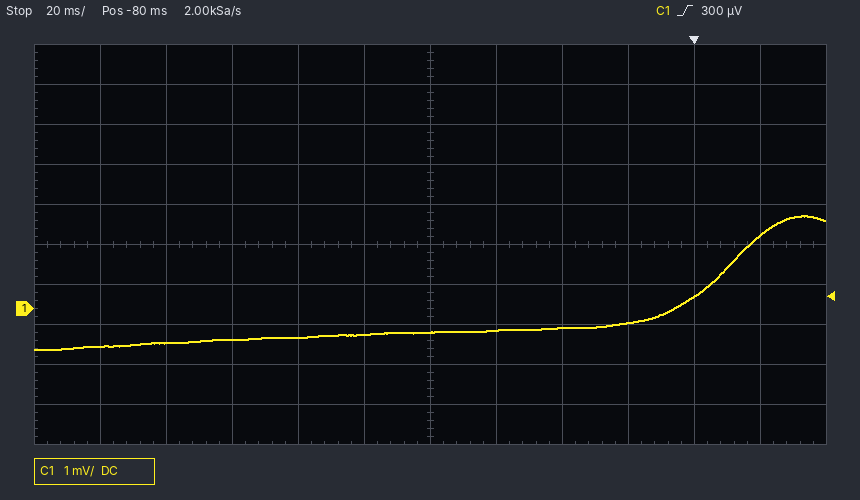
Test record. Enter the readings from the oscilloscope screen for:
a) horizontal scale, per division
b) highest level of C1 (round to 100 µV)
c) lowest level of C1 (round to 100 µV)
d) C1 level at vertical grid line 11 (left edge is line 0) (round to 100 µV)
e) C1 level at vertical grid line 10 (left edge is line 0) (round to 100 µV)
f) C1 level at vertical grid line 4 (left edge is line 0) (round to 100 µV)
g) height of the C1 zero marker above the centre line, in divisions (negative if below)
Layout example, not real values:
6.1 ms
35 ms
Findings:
20 ms
2.3 mV
-1.0 mV
1.8 mV
300 µV
-700 µV
-1.6 div
